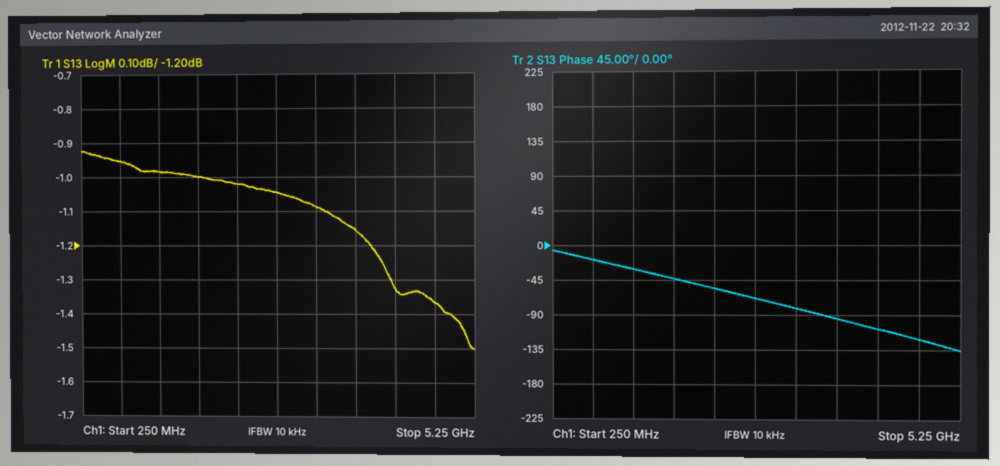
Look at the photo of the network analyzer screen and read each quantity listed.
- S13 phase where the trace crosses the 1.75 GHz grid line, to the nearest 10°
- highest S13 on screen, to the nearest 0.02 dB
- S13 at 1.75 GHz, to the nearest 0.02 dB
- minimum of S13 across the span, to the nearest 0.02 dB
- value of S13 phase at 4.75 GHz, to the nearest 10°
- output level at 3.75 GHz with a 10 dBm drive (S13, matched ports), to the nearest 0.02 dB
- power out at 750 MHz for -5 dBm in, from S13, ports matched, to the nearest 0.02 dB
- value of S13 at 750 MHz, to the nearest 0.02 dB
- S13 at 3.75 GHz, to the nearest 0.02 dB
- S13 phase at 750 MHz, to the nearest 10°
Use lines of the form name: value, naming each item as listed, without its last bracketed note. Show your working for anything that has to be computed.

S13 phase where the trace crosses the 1.75 GHz grid line, to the nearest 10°: -40°
highest S13 on screen, to the nearest 0.02 dB: -0.92 dB
S13 at 1.75 GHz, to the nearest 0.02 dB: -1.00 dB
minimum of S13 across the span, to the nearest 0.02 dB: -1.50 dB
value of S13 phase at 4.75 GHz, to the nearest 10°: -120°
output level at 3.75 GHz with a 10 dBm drive (S13, matched ports), to the nearest 0.02 dB: 10 dBm + (-1.16 dB) = 8.84 dBm
power out at 750 MHz for -5 dBm in, from S13, ports matched, to the nearest 0.02 dB: -5 dBm + (-0.96 dB) = -5.96 dBm
value of S13 at 750 MHz, to the nearest 0.02 dB: -0.96 dB
S13 at 3.75 GHz, to the nearest 0.02 dB: -1.16 dB
S13 phase at 750 MHz, to the nearest 10°: -20°
